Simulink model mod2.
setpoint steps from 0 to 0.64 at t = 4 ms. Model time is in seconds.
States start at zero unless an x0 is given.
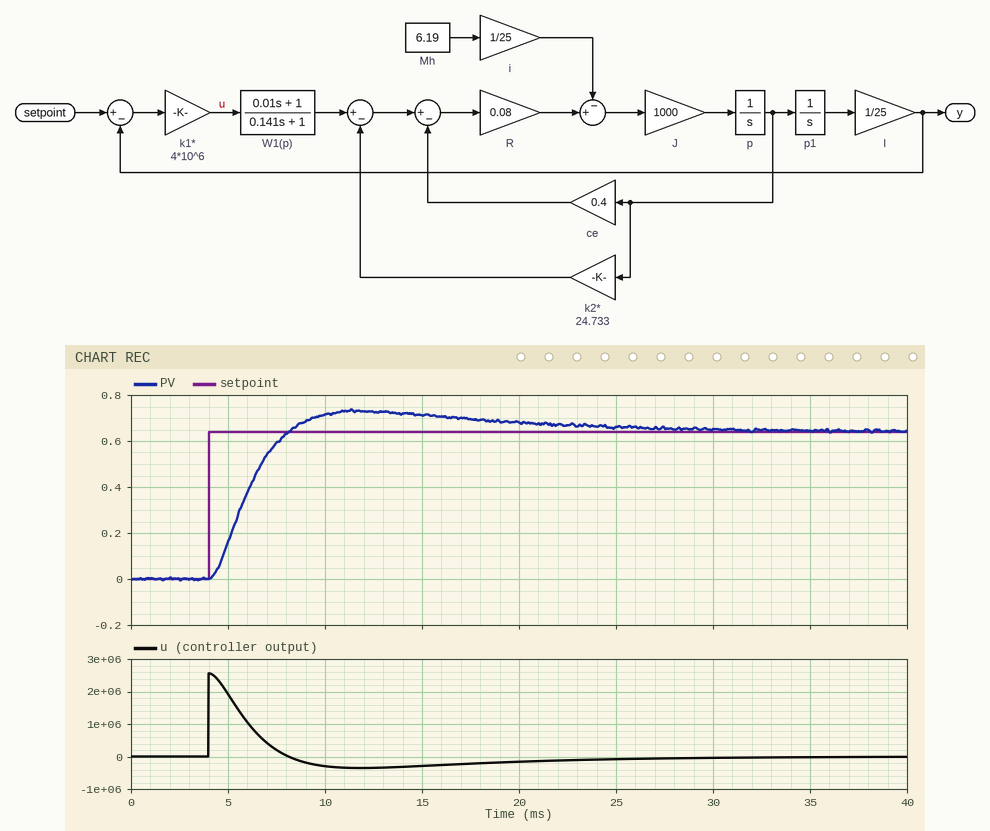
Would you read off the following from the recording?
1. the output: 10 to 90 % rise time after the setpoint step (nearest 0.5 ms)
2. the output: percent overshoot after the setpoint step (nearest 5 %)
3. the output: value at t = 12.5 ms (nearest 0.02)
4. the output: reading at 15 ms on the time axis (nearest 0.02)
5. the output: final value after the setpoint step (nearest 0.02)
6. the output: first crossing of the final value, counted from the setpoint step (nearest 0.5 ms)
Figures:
3.0 ms
15 %
0.72
0.72
0.64
4.0 ms
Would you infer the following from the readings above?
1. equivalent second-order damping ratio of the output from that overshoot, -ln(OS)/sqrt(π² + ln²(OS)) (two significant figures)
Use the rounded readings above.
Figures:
0.52
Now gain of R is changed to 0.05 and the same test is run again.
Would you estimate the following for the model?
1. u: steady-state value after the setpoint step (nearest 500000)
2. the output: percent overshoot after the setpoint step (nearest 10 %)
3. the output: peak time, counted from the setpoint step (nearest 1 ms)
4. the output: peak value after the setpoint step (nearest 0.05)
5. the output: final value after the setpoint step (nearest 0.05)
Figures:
0
20 %
7 ms
0.75
0.65
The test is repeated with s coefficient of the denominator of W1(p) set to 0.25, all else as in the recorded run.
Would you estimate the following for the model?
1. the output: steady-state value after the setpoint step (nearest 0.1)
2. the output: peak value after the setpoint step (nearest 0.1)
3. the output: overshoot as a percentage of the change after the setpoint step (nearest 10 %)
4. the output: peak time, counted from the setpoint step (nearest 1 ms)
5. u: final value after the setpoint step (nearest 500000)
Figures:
0.6
0.8
20 %
13 ms
0
